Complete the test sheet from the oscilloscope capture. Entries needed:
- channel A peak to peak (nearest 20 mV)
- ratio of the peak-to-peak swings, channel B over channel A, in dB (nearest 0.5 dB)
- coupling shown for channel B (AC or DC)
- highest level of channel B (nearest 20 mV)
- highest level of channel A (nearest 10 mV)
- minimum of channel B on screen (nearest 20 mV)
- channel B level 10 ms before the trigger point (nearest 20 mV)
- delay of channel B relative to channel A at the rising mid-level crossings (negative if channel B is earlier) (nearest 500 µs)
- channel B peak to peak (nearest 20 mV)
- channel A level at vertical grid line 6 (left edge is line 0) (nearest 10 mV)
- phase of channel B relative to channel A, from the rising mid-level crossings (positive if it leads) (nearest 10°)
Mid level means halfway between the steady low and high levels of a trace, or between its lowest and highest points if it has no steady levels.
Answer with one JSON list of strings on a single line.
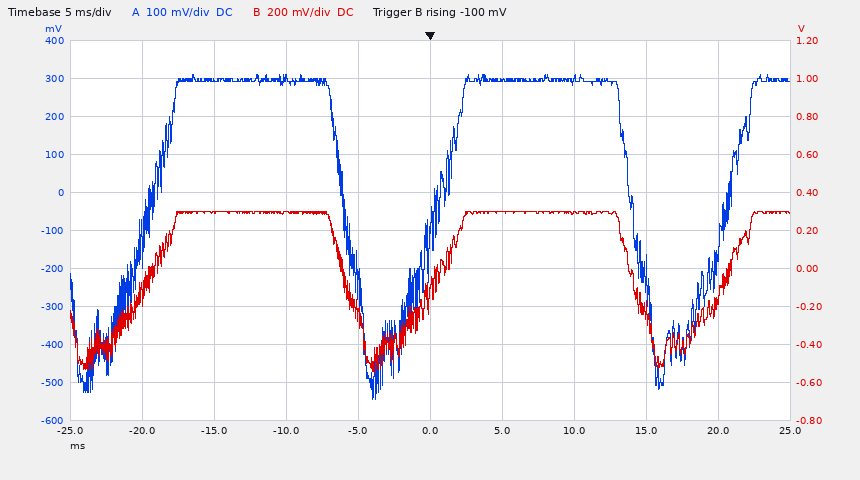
["860 mV", "0.0 dB", "DC", "300 mV", "310 mV", "-560 mV", "300 mV", "0.0 ms", "860 mV", "300 mV", "0°"]
